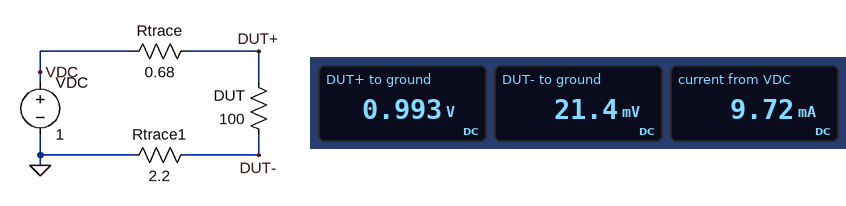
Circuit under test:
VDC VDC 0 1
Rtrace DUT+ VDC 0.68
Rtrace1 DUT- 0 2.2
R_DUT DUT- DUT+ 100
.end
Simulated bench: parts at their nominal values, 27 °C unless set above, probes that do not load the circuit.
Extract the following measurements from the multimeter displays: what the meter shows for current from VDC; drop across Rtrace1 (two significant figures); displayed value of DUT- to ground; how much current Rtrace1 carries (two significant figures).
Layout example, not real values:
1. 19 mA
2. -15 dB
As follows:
1. 9.72 mA
2. 21 mV
3. 21.4 mV
4. 9.7 mA
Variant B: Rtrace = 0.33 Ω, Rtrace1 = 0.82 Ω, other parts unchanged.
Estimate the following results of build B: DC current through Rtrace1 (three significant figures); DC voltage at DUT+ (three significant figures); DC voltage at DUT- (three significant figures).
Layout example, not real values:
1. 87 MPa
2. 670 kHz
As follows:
1. 9.89 mA
2. 997 mV
3. 8.11 mV
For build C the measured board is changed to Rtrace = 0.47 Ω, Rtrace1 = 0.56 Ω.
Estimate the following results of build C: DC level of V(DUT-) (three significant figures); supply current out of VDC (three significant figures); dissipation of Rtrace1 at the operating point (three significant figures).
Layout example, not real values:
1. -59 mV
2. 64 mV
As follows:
1. 5.54 mV
2. 9.90 mA
3. 54.9 µW
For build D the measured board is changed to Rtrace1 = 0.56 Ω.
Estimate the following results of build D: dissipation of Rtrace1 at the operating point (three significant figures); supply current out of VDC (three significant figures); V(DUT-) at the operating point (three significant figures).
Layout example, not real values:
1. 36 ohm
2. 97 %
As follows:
1. 54.6 µW
2. 9.88 mA
3. 5.53 mV
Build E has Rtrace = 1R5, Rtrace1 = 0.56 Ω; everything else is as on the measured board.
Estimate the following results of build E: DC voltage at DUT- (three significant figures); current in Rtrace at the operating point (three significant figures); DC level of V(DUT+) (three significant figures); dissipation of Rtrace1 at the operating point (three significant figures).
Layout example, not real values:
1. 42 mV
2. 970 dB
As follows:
1. 5.49 mV
2. 9.80 mA
3. 985 mV
4. 53.8 µW
